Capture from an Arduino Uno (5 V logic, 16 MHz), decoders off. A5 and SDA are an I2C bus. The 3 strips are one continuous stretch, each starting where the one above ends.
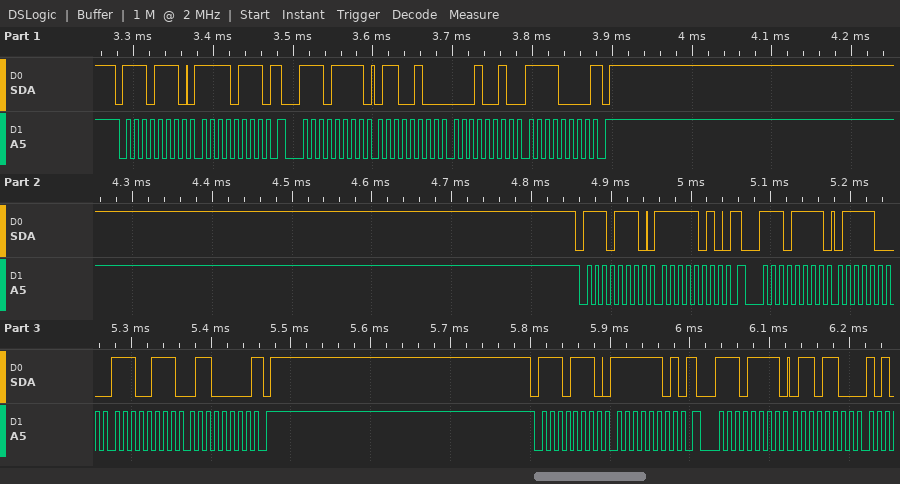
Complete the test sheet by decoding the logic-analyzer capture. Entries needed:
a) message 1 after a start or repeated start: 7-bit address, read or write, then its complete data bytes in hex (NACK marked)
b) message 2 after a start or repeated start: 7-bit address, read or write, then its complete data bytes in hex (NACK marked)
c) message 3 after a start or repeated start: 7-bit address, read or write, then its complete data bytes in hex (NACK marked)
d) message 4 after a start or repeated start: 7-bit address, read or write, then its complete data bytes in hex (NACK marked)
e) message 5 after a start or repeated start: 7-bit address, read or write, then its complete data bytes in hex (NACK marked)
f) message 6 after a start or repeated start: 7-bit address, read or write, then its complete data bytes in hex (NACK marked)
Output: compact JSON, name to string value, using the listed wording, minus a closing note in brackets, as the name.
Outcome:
{"message 1 after a start or repeated start: 7-bit address, read or write, then its complete data bytes in hex": "0x77 write: F7", "message 2 after a start or repeated start: 7-bit address, read or write, then its complete data bytes in hex": "0x77 read: 64 12 F0 NACK", "message 3 after a start or repeated start: 7-bit address, read or write, then its complete data bytes in hex": "0x77 write: FA", "message 4 after a start or repeated start: 7-bit address, read or write, then its complete data bytes in hex": "0x77 read: 78 E7 60 NACK", "message 5 after a start or repeated start: 7-bit address, read or write, then its complete data bytes in hex": "0x77 write: FD", "message 6 after a start or repeated start: 7-bit address, read or write, then its complete data bytes in hex": "0x77 read: 6C"}
